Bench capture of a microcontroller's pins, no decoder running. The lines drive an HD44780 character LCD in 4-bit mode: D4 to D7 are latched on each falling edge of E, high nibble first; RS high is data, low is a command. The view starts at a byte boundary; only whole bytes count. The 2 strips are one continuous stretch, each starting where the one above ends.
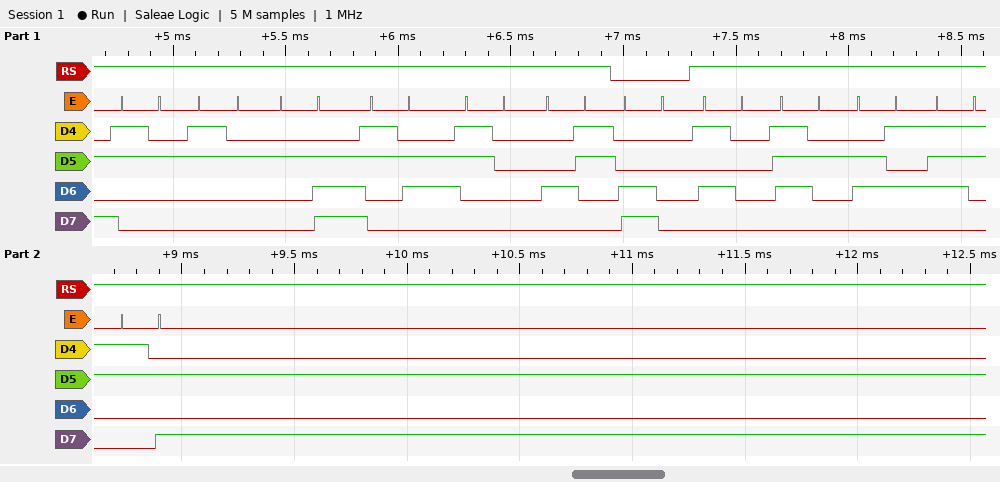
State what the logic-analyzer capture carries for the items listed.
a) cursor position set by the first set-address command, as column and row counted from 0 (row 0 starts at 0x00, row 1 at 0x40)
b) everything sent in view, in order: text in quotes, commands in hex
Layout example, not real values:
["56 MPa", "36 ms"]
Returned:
["column 0, row 1", "\"22.60C\" 0xC0 \"Pres:\""]
